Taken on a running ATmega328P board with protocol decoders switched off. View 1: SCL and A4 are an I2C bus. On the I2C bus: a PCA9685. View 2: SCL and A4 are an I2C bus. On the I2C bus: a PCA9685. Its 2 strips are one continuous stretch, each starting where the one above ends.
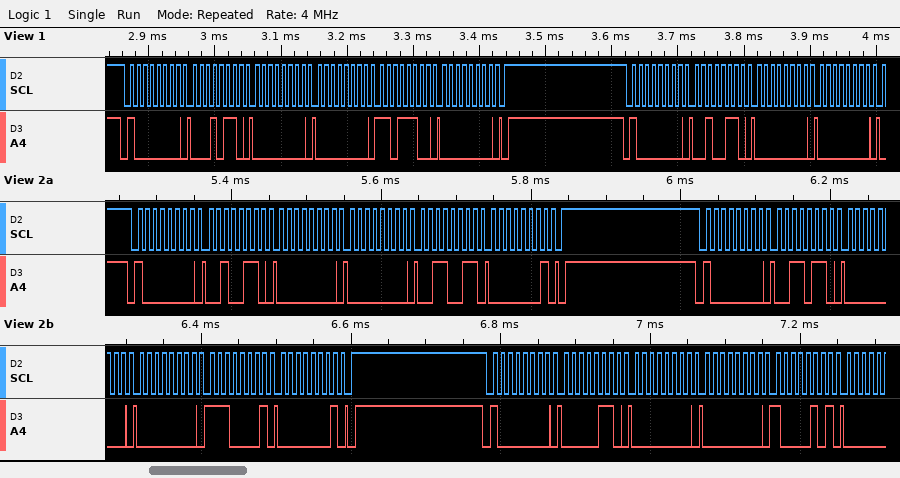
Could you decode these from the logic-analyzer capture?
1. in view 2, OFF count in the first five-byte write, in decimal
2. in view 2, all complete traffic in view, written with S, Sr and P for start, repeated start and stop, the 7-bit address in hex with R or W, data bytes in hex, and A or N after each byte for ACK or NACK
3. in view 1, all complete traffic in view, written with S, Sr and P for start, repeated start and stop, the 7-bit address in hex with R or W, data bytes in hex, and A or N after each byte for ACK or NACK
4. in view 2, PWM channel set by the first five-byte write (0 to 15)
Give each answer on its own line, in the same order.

307
S 40W A 26 A 00 A 00 A 33 A 01 A P S 40W A 36 A 00 A 00 A E1 A 01 A P S 40W A 06 A 00 A 00 A 85 A
S 40W A 16 A 00 A 00 A DC A 00 A P S 40W A 26 A 00 A 00 A
8
